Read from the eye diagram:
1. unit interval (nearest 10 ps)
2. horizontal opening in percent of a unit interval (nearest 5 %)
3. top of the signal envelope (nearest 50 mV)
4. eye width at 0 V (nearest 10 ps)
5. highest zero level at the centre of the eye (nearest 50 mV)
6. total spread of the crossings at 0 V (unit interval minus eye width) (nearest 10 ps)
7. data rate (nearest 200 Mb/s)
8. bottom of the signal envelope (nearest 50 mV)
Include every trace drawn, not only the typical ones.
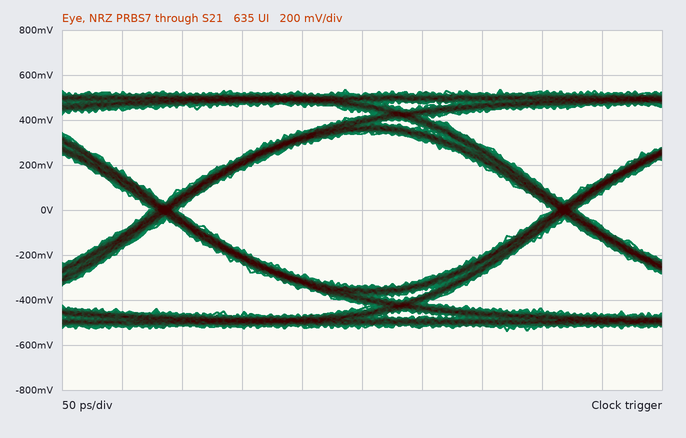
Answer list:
330 ps
95 %
550 mV
310 ps
-350 mV
20 ps
3.0 Gb/s
-550 mV
